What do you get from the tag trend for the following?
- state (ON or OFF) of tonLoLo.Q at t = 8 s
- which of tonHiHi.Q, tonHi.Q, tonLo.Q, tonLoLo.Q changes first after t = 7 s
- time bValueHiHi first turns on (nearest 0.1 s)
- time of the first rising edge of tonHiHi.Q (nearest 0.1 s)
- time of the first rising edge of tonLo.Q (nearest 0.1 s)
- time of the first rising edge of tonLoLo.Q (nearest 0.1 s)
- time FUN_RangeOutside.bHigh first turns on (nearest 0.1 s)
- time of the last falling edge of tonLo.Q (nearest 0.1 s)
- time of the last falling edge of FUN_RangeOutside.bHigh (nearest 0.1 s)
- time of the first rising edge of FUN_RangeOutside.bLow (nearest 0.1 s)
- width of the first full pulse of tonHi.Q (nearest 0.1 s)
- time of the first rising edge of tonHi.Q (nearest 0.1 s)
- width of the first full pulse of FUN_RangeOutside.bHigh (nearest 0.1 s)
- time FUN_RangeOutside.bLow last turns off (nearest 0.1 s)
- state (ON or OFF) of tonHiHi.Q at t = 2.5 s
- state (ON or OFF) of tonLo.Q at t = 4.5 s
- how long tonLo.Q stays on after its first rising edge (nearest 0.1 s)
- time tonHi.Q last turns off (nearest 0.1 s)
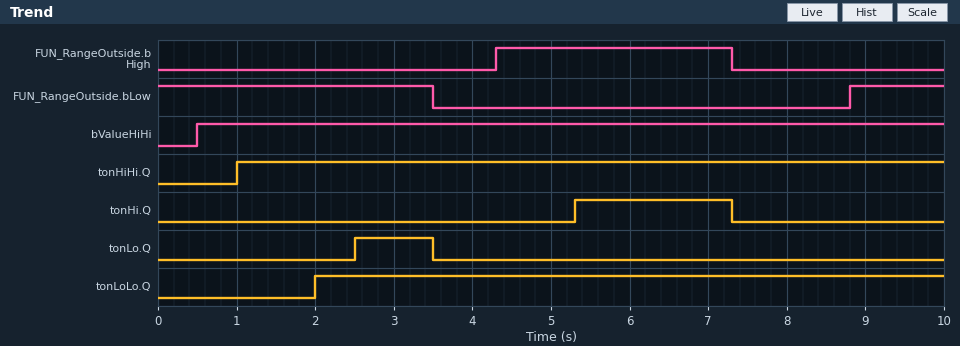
ON
tonHi.Q
0.5 s
1.0 s
2.5 s
2.0 s
4.3 s
3.5 s
7.3 s
8.8 s
2.0 s
5.3 s
3.0 s
3.5 s
ON
OFF
1.0 s
7.3 s
